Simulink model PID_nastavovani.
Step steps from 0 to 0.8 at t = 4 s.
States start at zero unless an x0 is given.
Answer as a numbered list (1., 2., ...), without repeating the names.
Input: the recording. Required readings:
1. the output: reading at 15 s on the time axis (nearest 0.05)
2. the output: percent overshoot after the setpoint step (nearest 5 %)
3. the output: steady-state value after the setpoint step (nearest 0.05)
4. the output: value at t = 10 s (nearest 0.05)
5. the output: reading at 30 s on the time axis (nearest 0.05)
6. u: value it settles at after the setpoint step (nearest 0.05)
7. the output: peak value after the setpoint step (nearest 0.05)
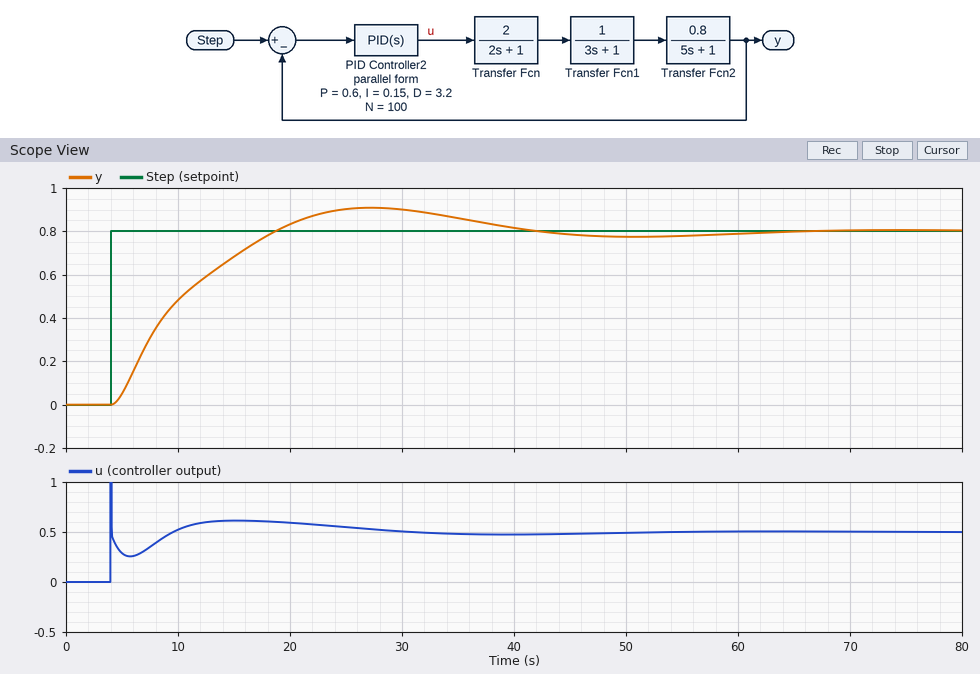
1. 0.70
2. 15 %
3. 0.80
4. 0.50
5. 0.90
6. 0.50
7. 0.90
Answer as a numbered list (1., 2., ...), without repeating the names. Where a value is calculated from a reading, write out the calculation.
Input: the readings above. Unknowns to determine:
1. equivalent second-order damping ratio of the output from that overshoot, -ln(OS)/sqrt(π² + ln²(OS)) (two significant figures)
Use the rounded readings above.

1. ln(0.15) = -1.897; 1.897 / sqrt(9.870 + 3.599) = 0.52
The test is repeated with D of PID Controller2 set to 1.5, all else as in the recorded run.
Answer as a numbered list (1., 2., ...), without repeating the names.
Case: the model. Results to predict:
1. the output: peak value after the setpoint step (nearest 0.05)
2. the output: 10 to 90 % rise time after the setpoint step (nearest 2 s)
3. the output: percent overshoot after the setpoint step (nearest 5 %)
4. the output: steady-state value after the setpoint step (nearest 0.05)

1. 0.95
2. 8 s
3. 20 %
4. 0.80
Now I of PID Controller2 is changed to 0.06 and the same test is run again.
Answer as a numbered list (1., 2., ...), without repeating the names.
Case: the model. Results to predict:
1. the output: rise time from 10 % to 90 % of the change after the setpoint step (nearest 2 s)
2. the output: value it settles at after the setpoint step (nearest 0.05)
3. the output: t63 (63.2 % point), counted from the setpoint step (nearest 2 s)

1. 26 s
2. 0.80
3. 10 s
